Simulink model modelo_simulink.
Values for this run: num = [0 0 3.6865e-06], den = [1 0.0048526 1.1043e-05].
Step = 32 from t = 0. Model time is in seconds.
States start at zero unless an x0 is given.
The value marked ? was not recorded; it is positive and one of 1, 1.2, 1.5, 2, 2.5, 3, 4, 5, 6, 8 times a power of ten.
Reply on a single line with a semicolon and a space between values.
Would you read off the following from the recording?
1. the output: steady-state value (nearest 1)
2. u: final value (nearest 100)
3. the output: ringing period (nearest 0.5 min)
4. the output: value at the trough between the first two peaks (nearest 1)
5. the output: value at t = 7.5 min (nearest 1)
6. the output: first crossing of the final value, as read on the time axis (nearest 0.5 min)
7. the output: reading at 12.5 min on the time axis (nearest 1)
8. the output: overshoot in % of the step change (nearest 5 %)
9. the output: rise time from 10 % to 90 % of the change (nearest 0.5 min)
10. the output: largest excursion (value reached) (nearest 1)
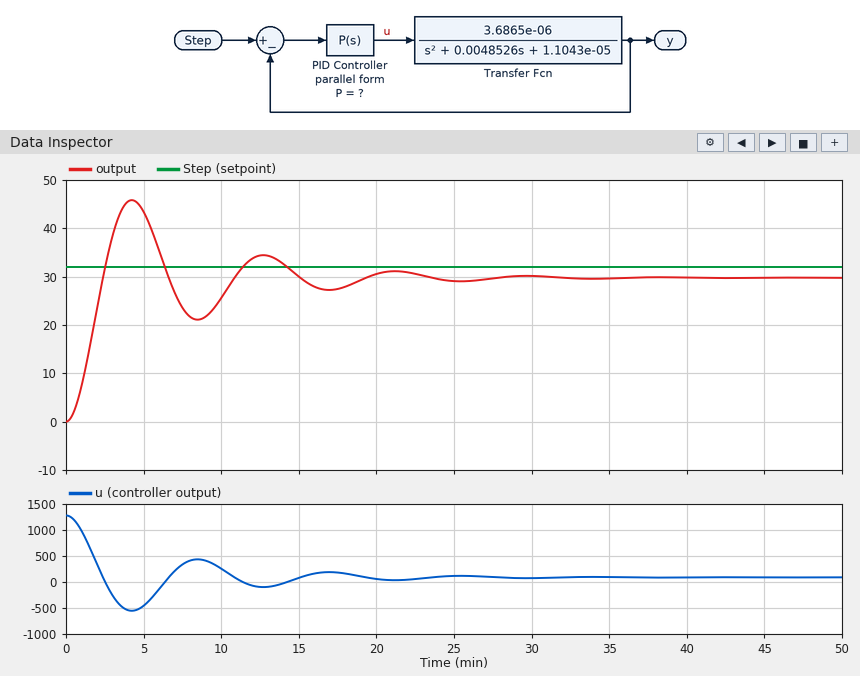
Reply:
30; 100; 8.5 min; 21; 24; 2.5 min; 34; 55 %; 1.5 min; 46
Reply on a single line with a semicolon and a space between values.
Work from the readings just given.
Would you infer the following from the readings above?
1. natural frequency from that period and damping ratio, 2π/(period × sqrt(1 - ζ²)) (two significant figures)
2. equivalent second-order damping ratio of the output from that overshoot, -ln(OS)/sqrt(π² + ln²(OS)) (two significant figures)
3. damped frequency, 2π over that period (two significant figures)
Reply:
0.75 rad/min; 0.19; 0.74 rad/min
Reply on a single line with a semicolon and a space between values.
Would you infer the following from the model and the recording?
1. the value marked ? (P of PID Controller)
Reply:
40
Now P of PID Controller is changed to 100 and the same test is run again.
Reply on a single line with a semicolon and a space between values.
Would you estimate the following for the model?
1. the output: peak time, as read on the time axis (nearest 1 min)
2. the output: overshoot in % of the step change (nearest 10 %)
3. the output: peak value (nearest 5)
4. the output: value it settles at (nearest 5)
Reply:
3 min; 70 %; 50; 30
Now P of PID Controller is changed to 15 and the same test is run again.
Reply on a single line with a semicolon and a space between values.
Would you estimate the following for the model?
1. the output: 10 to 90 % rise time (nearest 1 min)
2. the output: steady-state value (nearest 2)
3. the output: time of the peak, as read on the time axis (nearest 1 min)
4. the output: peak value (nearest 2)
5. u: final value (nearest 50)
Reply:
3 min; 26; 7 min; 36; 100
